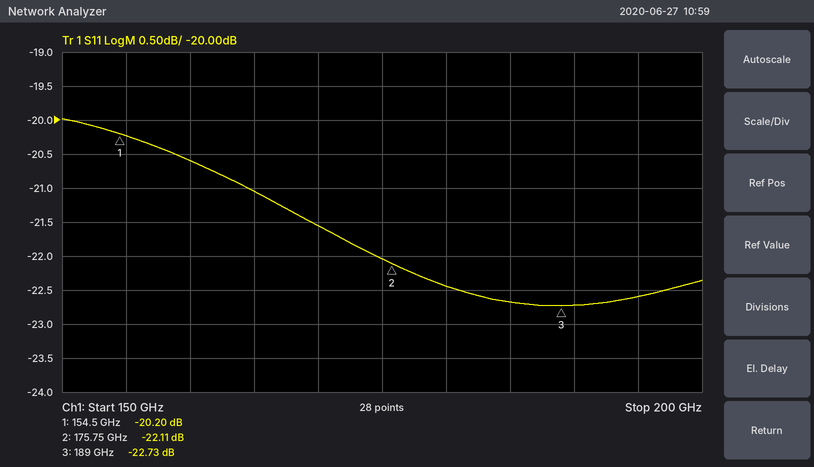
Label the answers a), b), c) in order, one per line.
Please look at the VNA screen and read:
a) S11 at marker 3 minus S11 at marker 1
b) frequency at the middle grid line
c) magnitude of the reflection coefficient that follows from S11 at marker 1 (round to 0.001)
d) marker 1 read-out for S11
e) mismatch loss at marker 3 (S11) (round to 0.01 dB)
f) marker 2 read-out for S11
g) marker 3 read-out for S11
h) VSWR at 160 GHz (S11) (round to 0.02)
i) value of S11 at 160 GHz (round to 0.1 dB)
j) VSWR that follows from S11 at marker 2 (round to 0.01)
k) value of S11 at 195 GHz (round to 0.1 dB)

a) -2.53 dB
b) 175 GHz
c) 0.098
d) -20.20 dB
e) 0.02 dB
f) -22.11 dB
g) -22.73 dB
h) 1.20
i) -20.6 dB
j) 1.17
k) -22.6 dB
